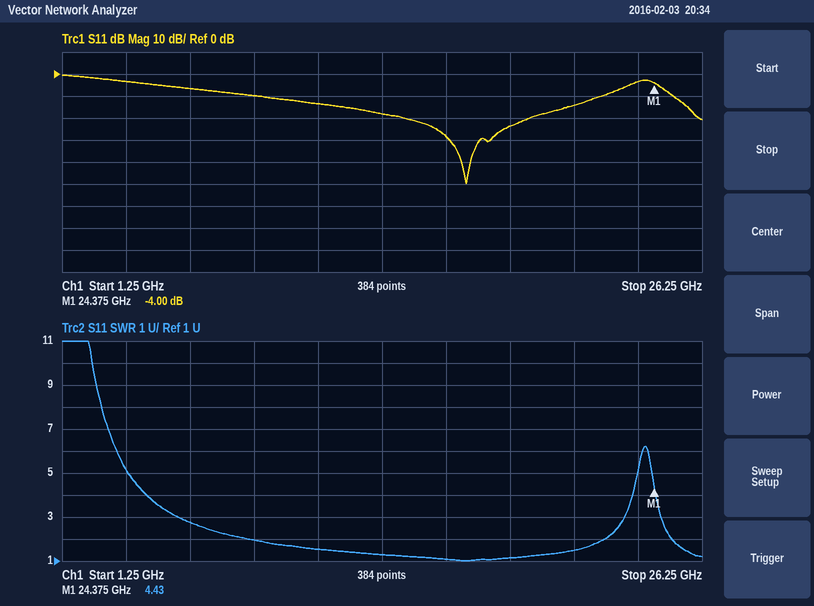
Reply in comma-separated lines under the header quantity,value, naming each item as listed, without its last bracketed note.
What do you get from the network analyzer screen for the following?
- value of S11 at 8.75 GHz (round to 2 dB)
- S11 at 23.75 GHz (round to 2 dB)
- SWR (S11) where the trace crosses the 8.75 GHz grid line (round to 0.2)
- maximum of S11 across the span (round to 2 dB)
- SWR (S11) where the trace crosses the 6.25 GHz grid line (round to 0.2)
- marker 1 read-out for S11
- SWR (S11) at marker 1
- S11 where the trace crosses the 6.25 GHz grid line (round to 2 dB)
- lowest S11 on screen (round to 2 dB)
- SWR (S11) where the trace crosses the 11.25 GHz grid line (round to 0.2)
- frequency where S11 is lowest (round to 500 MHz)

quantity,value
value of S11 at 8.75 GHz,-10 dB
S11 at 23.75 GHz,-4 dB
SWR (S11) where the trace crosses the 8.75 GHz grid line,2.0
maximum of S11 across the span,0 dB
SWR (S11) where the trace crosses the 6.25 GHz grid line,2.8
marker 1 read-out for S11,-4.00 dB
SWR (S11) at marker 1,4.43
S11 where the trace crosses the 6.25 GHz grid line,-6 dB
lowest S11 on screen,-50 dB
SWR (S11) where the trace crosses the 11.25 GHz grid line,1.6
frequency where S11 is lowest,17.0 GHz
